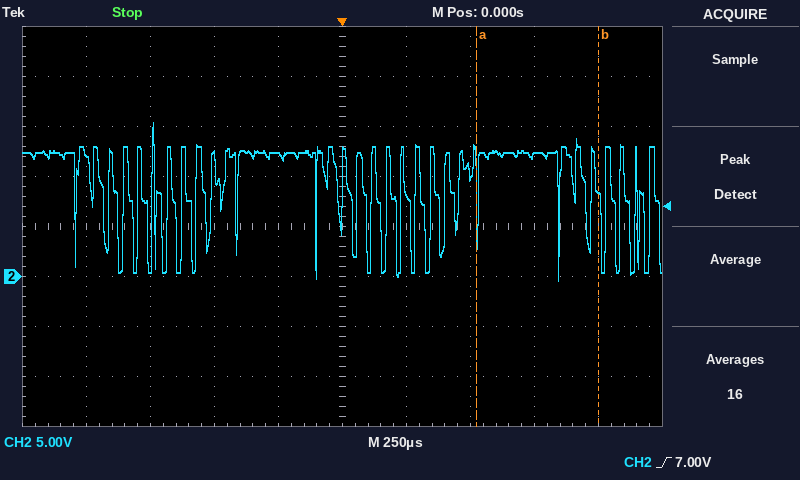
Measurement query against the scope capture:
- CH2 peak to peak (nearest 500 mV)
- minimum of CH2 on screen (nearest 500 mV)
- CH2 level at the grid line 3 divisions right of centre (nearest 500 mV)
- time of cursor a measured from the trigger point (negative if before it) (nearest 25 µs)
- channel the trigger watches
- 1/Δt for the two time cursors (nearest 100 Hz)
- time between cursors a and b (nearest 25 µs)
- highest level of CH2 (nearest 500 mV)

16.0 V
-500 mV
12.0 V
+525 µs
CH2
2.1 kHz
475 µs
15.5 V
